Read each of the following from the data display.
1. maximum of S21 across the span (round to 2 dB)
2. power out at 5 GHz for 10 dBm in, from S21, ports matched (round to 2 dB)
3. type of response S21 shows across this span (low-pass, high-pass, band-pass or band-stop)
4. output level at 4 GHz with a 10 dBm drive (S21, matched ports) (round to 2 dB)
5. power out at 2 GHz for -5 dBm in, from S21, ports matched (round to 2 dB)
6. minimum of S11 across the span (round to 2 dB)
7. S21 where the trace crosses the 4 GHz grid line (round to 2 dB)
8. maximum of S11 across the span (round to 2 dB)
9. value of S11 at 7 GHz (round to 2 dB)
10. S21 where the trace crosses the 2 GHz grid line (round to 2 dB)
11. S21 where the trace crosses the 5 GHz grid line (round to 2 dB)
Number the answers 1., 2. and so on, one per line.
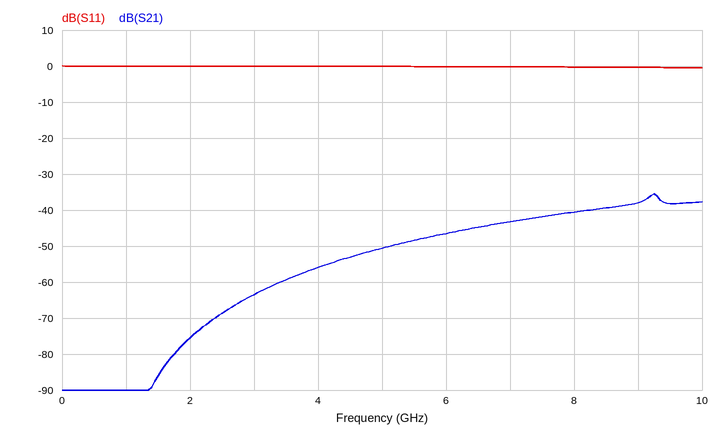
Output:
1. -36 dB
2. -40 dBm
3. high-pass
4. -46 dBm
5. -80 dBm
6. 0 dB
7. -56 dB
8. 0 dB
9. 0 dB
10. -76 dB
11. -50 dB
